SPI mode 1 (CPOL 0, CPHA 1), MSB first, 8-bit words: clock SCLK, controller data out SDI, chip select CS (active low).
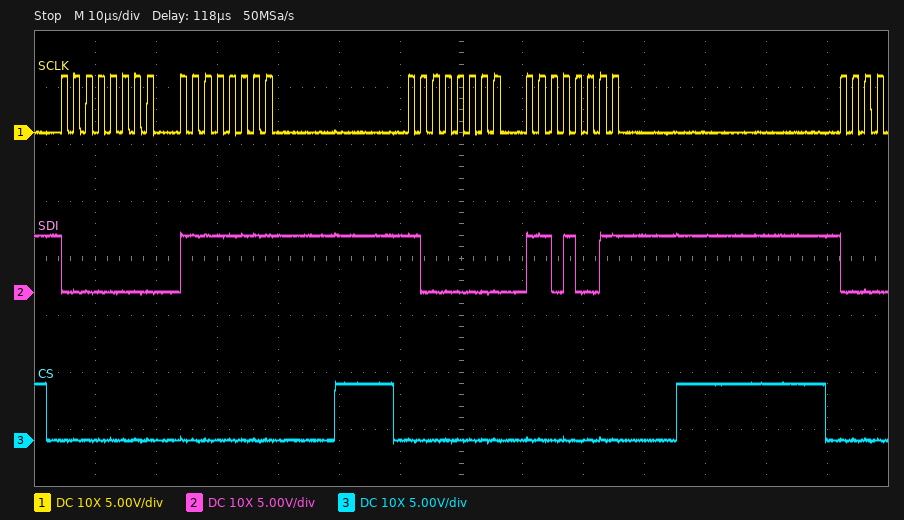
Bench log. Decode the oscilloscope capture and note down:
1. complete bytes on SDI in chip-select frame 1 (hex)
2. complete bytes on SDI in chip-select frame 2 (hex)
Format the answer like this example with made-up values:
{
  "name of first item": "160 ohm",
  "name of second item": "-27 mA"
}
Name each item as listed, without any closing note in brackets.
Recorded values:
{
  "complete bytes on SDI in chip-select frame 1": "00 FF",
  "complete bytes on SDI in chip-select frame 2": "80 D3"
}
